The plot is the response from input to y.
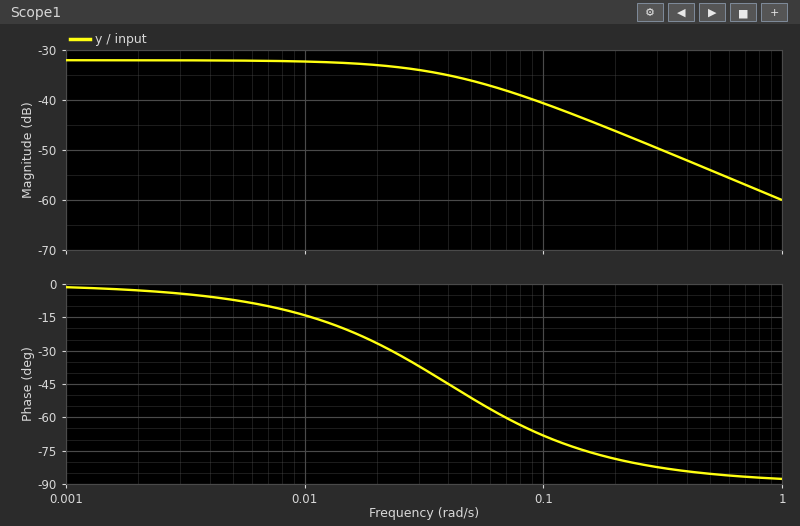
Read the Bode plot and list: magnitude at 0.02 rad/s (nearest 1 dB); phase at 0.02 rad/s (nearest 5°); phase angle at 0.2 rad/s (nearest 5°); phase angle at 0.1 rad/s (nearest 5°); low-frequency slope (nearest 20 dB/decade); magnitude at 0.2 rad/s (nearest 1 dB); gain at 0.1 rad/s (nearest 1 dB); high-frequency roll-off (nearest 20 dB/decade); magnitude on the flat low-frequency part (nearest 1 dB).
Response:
-33 dB
-25°
-80°
-70°
0 dB/decade
-46 dB
-41 dB
-20 dB/decade
-32 dB
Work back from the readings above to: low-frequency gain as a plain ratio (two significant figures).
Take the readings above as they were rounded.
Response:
0.025
